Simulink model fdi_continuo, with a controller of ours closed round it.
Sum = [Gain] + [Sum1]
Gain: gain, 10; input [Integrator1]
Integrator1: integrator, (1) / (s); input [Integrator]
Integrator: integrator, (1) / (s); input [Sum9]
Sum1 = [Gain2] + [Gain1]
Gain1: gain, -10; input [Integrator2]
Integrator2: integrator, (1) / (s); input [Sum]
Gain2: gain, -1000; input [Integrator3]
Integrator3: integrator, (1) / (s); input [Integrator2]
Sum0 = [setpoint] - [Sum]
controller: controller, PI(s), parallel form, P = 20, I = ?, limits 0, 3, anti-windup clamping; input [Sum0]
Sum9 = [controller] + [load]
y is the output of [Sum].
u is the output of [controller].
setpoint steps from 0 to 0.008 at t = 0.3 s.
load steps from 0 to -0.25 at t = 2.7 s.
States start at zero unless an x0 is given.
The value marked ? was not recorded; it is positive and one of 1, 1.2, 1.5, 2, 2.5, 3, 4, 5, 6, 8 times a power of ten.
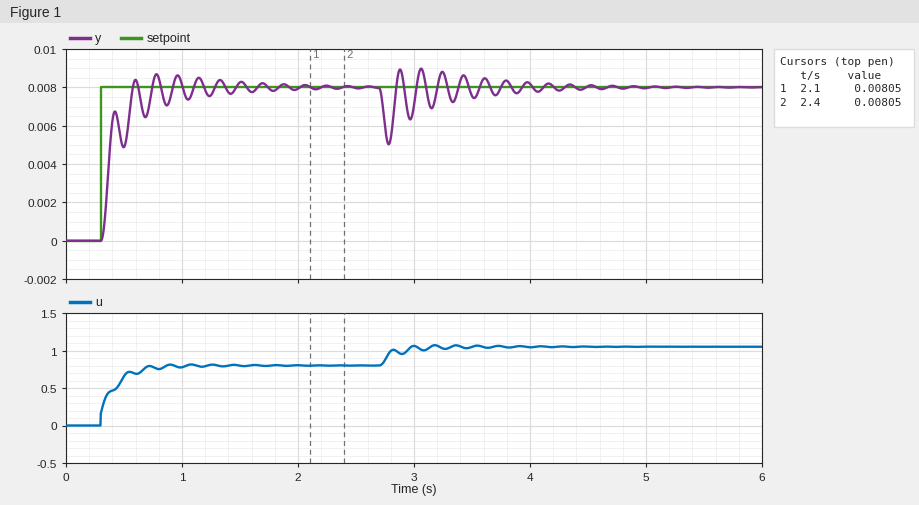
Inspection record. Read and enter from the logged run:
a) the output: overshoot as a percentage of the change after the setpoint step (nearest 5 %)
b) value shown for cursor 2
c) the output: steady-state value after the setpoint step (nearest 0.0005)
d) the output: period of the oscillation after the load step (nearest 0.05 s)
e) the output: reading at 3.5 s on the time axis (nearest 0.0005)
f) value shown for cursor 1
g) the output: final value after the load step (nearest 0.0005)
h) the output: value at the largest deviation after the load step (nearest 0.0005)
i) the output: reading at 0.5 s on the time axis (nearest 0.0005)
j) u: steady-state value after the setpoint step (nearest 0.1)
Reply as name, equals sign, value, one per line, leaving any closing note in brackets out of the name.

the output: overshoot as a percentage of the change after the setpoint step = 10 %
value shown for cursor 2 = 0.00805
the output: steady-state value after the setpoint step = 0.0080
the output: period of the oscillation after the load step = 0.20 s
the output: reading at 3.5 s on the time axis = 0.0075
value shown for cursor 1 = 0.00805
the output: final value after the load step = 0.0080
the output: value at the largest deviation after the load step = 0.0050
the output: reading at 0.5 s on the time axis = 0.0050
u: steady-state value after the setpoint step = 0.8
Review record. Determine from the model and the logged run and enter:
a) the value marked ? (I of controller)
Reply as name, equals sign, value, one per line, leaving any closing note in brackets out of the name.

the value marked ? = 800
